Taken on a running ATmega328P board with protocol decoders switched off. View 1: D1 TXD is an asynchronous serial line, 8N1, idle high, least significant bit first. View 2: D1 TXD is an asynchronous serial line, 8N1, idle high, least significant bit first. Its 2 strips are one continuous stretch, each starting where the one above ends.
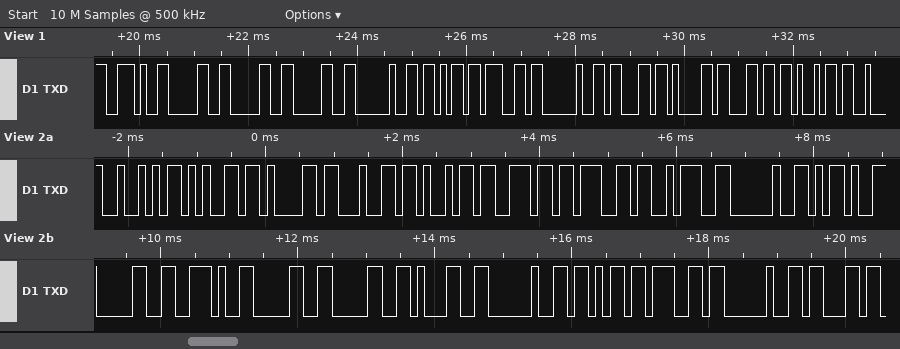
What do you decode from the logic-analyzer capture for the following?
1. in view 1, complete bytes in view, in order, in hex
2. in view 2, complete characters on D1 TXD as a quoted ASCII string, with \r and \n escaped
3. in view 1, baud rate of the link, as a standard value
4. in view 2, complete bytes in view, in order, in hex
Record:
0x2E 0x30 0x30 0x30 0x20 0x6B 0x67 0x20 0x63 0x61 0x6C 0x69
"Reading: -0.001 kg c"
9600 baud
52 65 61 64 69 6E 67 3A 20 2D 30 2E 30 30 31 20 6B 67 20 63
